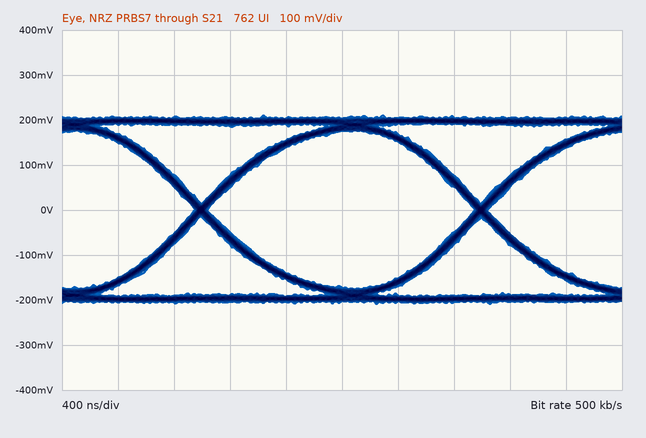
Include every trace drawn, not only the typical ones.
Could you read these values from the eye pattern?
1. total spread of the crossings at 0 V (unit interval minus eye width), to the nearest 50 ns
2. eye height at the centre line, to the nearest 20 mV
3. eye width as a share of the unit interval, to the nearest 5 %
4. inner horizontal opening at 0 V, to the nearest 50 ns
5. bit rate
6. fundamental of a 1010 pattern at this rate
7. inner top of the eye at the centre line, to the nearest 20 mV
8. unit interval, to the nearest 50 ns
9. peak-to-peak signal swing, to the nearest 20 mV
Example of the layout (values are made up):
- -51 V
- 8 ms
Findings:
- 100 ns
- 340 mV
- 95 %
- 1.90 µs
- 500 kb/s
- 250 kHz
- 180 mV
- 2.00 µs
- 420 mV
